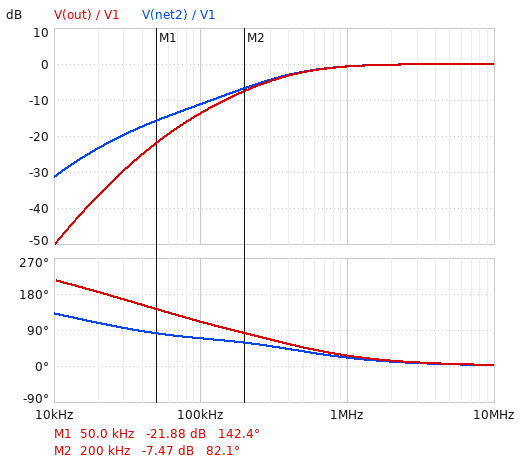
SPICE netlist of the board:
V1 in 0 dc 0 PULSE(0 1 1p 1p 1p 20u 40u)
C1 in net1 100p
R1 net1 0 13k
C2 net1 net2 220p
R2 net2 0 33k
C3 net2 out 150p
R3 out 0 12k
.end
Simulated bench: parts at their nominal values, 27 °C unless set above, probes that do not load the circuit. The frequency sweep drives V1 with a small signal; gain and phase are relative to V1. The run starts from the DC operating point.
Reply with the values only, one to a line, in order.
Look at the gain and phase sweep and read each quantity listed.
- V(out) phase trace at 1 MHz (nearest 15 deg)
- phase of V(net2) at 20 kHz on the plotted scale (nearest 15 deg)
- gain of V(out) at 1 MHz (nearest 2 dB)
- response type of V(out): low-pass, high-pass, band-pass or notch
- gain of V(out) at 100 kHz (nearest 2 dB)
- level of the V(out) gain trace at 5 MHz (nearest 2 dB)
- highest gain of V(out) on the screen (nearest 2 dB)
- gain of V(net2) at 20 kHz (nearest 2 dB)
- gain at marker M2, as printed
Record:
30 deg
105 deg
0 dB
high-pass
-14 dB
0 dB
0 dB
-24 dB
-7.47 dB
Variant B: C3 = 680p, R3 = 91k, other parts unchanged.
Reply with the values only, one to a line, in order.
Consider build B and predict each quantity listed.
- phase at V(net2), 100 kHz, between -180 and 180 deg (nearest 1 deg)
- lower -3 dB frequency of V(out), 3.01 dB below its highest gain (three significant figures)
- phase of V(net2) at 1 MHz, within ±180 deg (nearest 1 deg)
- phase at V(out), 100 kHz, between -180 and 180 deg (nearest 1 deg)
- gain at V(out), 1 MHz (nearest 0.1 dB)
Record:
74 deg
202 kHz
12 deg
75 deg
-0.2 dB
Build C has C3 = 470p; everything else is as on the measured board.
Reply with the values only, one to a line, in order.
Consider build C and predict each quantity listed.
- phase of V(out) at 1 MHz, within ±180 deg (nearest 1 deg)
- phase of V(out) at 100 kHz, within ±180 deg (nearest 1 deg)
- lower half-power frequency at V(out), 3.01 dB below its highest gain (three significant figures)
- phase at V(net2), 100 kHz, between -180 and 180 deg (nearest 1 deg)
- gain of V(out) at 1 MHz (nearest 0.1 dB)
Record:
23 deg
98 deg
376 kHz
82 deg
-0.6 dB
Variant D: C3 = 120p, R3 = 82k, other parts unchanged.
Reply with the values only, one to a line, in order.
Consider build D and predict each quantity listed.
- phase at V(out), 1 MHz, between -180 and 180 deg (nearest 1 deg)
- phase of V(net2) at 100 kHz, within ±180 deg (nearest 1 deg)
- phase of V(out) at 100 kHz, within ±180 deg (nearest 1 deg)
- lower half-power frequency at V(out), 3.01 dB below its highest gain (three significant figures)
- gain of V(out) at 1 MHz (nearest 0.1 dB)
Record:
13 deg
73 deg
82 deg
207 kHz
-0.2 dB
